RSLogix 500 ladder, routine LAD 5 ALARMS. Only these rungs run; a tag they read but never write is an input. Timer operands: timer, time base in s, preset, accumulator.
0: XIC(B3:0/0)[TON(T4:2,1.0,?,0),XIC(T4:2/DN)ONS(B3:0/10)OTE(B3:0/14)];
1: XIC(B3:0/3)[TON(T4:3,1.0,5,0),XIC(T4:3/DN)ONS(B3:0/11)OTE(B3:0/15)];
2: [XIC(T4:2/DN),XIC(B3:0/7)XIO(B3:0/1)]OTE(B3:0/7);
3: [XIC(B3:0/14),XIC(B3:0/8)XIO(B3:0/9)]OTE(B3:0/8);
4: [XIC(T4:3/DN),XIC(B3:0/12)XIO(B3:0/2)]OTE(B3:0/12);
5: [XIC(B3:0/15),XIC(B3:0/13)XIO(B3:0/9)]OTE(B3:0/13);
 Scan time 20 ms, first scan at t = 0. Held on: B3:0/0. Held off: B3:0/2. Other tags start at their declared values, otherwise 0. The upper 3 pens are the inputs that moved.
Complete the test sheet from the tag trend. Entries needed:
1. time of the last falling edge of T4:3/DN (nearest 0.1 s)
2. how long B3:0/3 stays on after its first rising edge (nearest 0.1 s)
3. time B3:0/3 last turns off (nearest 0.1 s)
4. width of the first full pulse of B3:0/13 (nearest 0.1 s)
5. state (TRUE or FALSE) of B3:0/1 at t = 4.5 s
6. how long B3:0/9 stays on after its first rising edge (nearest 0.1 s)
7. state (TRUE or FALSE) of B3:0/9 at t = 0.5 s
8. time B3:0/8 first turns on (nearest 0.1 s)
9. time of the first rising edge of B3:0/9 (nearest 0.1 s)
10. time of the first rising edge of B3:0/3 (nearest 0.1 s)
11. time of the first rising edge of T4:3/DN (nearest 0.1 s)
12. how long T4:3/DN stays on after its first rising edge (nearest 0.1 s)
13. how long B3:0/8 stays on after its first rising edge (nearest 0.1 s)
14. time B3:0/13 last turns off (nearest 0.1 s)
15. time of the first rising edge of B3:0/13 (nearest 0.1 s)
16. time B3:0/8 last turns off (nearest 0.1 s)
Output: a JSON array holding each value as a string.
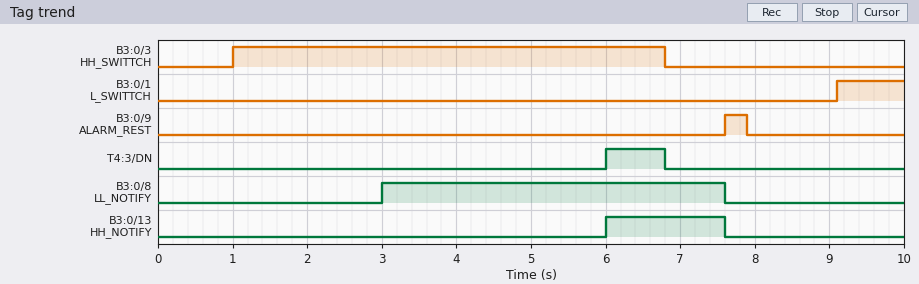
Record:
["6.8 s", "5.8 s", "6.8 s", "1.6 s", "FALSE", "0.3 s", "FALSE", "3.0 s", "7.6 s", "1.0 s", "6.0 s", "0.8 s", "4.6 s", "7.6 s", "6.0 s", "7.6 s"]
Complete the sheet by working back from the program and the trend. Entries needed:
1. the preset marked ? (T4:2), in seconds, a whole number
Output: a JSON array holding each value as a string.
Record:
["3 s"]
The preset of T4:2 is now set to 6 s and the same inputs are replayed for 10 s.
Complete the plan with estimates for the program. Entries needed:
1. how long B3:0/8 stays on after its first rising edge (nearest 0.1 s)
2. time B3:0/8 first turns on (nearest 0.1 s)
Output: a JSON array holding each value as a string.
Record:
["1.6 s", "6.0 s"]
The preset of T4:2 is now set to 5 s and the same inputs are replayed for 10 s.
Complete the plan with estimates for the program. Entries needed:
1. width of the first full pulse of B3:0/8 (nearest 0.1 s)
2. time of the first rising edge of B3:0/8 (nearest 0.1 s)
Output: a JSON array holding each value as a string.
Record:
["2.6 s", "5.0 s"]
